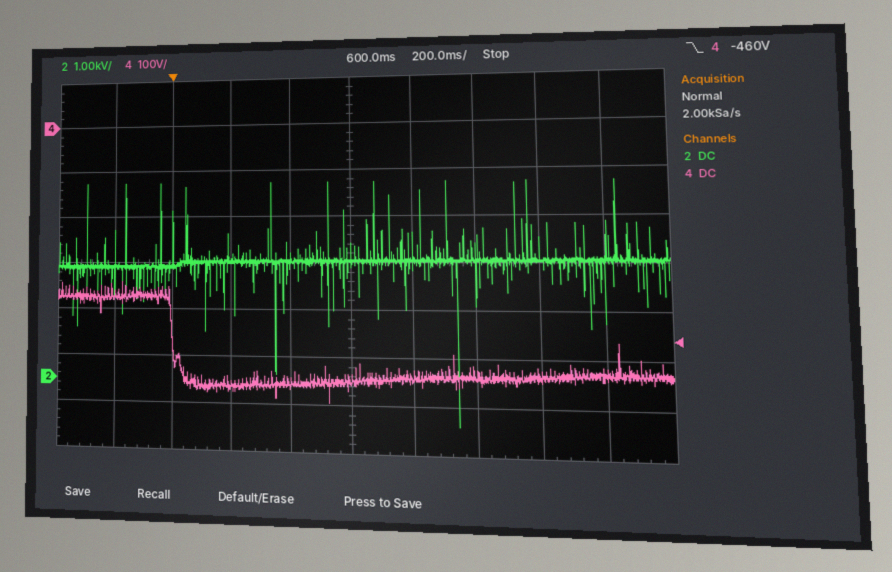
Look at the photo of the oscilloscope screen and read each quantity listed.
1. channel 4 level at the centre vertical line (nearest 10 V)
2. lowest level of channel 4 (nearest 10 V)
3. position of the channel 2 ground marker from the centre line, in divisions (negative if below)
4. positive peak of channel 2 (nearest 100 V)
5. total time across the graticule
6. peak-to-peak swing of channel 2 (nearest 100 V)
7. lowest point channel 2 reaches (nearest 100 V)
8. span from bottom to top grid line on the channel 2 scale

-550 V
-590 V
-2.5 div
4.2 kV
2 s
5.1 kV
-900 V
8 kV
